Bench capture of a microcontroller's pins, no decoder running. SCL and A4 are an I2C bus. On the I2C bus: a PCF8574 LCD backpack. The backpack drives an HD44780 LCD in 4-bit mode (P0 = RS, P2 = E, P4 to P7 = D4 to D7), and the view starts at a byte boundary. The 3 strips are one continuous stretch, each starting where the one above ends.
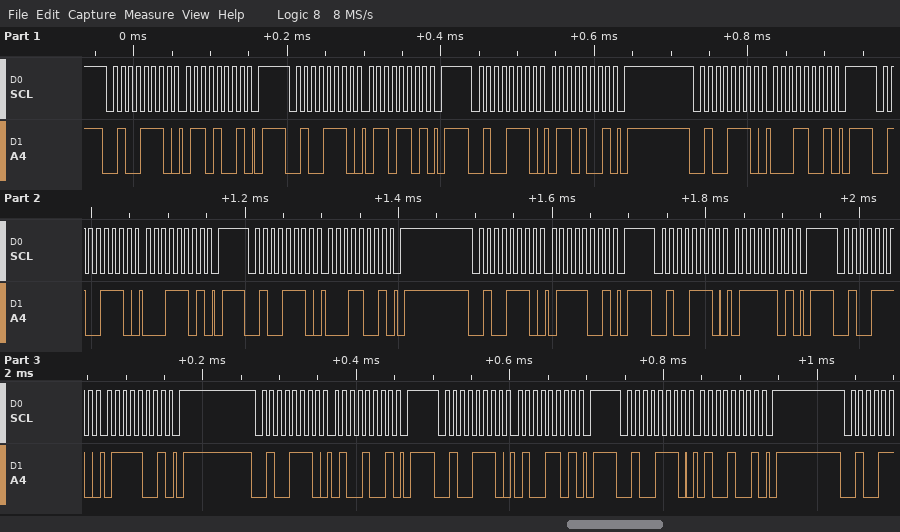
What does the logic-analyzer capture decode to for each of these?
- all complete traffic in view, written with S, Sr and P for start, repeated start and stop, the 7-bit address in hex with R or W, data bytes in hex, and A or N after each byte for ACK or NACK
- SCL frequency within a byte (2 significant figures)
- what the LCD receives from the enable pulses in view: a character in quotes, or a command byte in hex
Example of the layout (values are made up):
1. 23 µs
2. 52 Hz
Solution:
1. S 27W A 69 A P S 27W A 6D A P S 27W A 69 A P S 27W A 19 A P S 27W A 1D A P S 27W A 19 A P S 27W A 79 A P S 27W A 7D A P S 27W A 79 A P S 27W A 49 A P S 27W A 4D A P S 27W A 49 A P
2. 100 kHz
3. 'a' 't'
